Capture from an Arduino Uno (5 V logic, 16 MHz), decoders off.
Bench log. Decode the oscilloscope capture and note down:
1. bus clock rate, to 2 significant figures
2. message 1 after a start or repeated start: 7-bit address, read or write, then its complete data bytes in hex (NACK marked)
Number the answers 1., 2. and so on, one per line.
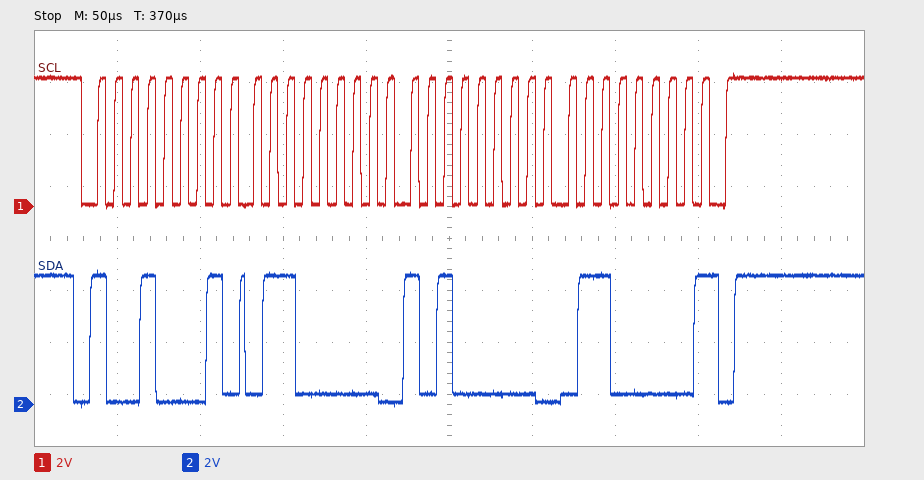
1. 100 kHz
2. 0x48 read: 60 A0 60 NACK
